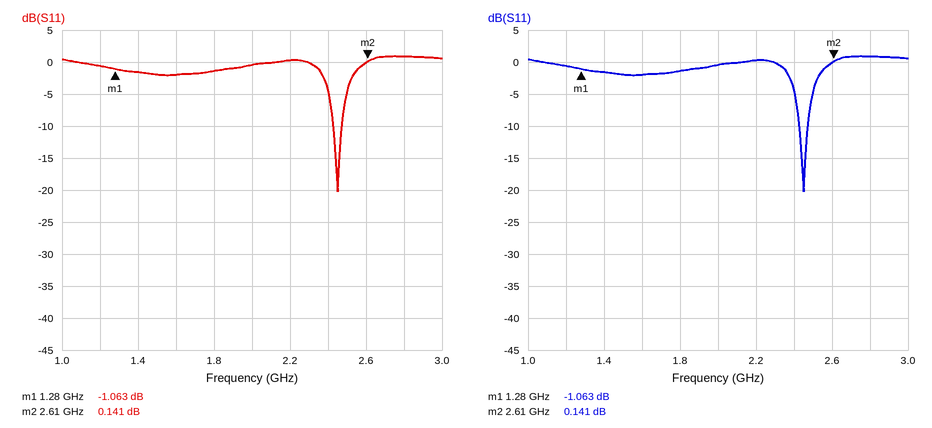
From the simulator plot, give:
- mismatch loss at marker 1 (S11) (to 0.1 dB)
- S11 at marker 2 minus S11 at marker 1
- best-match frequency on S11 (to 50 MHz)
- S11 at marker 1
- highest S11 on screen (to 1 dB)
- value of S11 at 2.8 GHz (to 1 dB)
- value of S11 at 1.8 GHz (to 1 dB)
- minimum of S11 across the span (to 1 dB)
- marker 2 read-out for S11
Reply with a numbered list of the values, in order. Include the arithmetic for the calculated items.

1. −10 log10(1 − 10^(-1.063/10)) ≈ 6.6 dB
2. 0.141 − (-1.063) = 1.204 dB
3. 2.45 GHz
4. -1.063 dB
5. 1 dB
6. 1 dB
7. -1 dB
8. -20 dB
9. 0.141 dB
